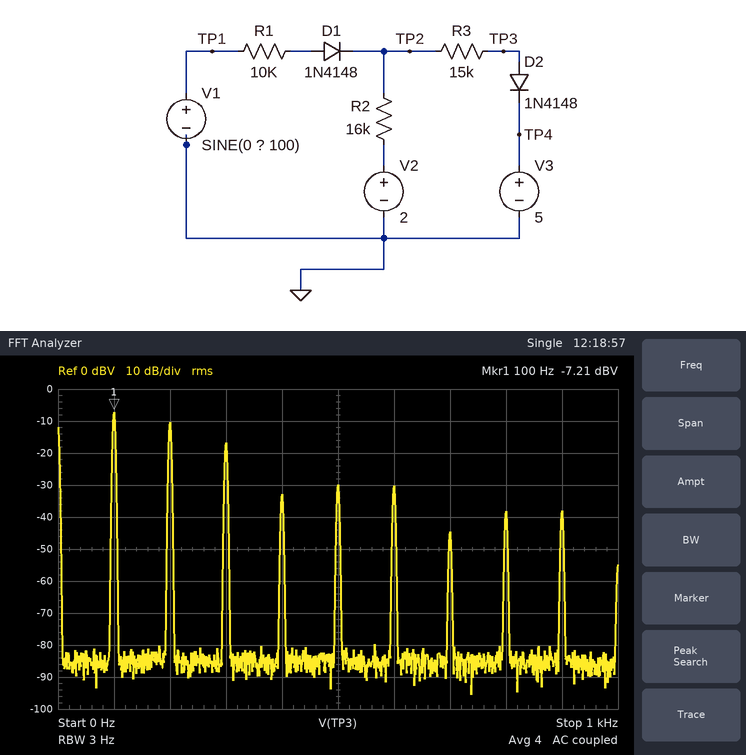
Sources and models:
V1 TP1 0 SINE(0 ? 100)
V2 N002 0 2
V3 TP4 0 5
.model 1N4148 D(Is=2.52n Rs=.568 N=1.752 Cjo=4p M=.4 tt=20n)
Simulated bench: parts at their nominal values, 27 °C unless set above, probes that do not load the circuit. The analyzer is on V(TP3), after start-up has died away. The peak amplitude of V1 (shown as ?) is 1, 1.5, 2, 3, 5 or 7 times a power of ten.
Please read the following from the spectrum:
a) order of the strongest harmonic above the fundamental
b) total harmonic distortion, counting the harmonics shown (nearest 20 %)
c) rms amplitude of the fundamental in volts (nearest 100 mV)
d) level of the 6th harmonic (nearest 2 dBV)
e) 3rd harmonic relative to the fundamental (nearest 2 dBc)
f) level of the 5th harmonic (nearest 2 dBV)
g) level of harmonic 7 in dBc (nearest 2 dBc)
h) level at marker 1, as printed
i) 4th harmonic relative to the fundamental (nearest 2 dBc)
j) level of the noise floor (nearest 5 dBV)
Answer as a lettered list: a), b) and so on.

a) 2
b) 80 %
c) 400 mV
d) -30 dBV
e) -10 dBc
f) -30 dBV
g) -38 dBc
h) -7.21 dBV
i) -26 dBc
j) -85 dBV
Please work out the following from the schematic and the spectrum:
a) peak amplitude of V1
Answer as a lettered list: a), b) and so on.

a) 5 V
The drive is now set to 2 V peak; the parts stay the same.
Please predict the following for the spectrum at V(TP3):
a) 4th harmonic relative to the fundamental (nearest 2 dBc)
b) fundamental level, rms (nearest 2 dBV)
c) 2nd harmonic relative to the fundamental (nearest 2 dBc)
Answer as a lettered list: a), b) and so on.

a) -22 dBc
b) -88 dBV
c) -16 dBc
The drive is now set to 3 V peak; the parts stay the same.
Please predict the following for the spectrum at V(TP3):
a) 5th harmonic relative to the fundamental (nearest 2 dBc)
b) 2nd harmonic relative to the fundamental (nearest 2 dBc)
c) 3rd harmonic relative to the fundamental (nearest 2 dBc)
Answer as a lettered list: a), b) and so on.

a) -12 dBc
b) -2 dBc
c) -4 dBc
